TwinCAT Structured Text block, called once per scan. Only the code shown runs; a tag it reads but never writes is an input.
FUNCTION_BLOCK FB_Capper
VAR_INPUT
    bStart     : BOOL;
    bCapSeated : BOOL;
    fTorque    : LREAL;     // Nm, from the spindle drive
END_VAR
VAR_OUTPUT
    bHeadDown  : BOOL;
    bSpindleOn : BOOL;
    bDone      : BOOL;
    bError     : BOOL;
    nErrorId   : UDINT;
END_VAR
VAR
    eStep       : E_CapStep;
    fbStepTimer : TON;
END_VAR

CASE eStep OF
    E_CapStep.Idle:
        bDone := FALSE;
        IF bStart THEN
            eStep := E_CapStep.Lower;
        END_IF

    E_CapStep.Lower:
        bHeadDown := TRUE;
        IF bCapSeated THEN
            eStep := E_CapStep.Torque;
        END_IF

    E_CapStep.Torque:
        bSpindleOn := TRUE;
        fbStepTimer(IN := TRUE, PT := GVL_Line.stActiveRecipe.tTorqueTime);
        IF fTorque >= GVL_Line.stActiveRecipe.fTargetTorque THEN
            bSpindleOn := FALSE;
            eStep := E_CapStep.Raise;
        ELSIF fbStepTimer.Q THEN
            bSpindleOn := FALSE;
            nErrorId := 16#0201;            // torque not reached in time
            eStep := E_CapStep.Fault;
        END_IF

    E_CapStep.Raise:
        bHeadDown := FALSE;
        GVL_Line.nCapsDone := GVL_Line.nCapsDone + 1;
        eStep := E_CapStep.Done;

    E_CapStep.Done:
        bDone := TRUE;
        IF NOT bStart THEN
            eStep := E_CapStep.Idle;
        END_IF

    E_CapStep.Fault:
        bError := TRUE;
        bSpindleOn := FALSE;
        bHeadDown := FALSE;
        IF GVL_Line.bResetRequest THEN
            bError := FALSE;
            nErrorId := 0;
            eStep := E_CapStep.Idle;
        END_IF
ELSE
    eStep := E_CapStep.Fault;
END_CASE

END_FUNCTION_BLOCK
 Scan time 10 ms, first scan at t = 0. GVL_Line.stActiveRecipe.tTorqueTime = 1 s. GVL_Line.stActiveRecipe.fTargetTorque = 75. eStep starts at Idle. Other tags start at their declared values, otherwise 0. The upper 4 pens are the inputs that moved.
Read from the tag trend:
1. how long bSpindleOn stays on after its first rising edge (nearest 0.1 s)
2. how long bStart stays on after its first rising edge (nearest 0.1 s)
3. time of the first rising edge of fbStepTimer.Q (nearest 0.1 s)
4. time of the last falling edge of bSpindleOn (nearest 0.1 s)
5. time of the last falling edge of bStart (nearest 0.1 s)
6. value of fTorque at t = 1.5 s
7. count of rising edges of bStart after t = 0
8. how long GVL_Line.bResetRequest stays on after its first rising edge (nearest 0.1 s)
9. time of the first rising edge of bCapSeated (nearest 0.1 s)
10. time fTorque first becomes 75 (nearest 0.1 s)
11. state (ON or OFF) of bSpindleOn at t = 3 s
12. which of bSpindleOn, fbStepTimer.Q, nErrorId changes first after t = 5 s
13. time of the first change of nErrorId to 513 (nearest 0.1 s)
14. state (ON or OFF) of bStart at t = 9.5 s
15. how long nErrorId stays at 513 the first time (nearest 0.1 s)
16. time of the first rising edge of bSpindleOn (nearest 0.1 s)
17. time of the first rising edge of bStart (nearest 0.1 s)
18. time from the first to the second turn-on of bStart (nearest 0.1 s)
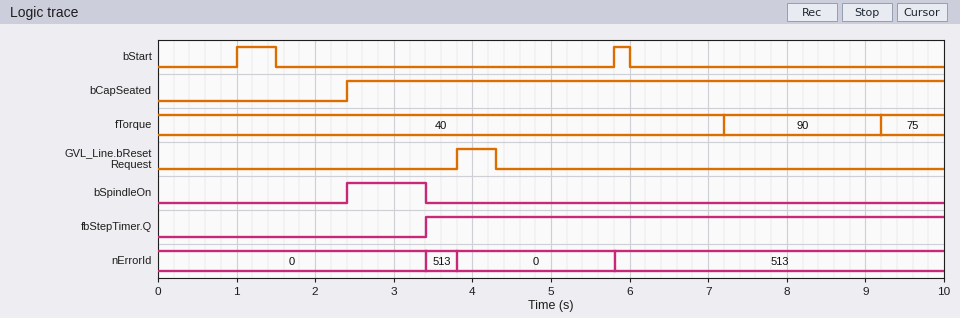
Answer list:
1.0 s
0.5 s
3.4 s
3.4 s
6.0 s
40
2
0.5 s
2.4 s
9.2 s
ON
nErrorId
3.4 s
OFF
0.4 s
2.4 s
1.0 s
4.8 s
